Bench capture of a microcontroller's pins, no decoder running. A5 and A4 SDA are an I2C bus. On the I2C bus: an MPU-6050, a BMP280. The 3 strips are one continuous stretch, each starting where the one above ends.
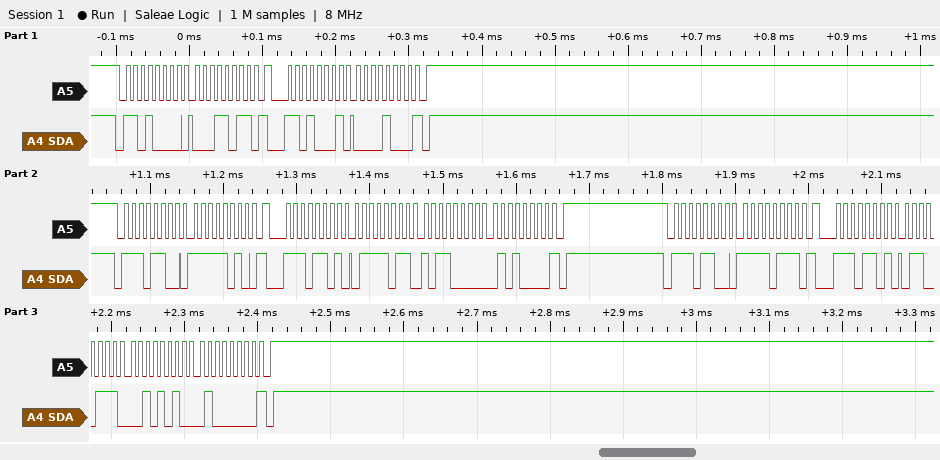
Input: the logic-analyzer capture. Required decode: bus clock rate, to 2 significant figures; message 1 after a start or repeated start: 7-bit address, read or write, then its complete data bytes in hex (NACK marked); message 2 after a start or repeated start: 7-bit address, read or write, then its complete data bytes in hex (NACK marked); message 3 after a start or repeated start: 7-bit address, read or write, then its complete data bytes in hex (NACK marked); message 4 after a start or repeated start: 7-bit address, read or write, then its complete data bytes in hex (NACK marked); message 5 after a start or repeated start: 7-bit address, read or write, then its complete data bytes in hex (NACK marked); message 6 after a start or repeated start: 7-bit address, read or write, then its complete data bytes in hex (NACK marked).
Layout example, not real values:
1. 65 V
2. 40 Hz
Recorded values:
1. 100 kHz
2. 0x68 write: 1B
3. 0x68 read: 08 NACK
4. 0x76 write: FA
5. 0x76 read: 7B B0 50 NACK
6. 0x76 write: F7
7. 0x76 read: 67 2A 40 NACK
